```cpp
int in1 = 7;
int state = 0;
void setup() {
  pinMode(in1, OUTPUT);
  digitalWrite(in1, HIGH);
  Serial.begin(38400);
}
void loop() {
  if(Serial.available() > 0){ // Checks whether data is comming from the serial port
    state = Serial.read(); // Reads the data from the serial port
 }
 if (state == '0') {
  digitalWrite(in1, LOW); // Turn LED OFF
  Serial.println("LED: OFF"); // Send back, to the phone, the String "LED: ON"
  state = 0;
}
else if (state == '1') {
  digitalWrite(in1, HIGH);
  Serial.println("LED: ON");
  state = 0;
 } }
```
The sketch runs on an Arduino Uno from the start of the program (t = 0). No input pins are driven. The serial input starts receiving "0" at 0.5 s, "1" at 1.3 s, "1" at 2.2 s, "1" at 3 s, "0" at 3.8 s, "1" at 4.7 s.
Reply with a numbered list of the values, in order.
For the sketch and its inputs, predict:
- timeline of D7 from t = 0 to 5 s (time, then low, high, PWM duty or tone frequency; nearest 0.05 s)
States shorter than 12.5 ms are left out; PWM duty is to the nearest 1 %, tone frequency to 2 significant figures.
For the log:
1. 0 s high; 0.5 s low; 1.3 s high; 3.8 s low; 4.7 s high
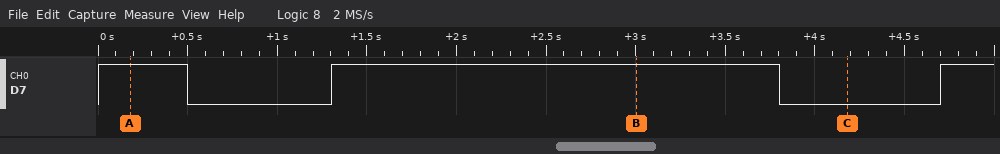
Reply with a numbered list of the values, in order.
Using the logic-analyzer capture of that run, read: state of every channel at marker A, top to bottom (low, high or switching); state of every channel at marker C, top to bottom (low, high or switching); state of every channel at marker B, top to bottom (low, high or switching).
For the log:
1. D7 high
2. D7 low
3. D7 high
